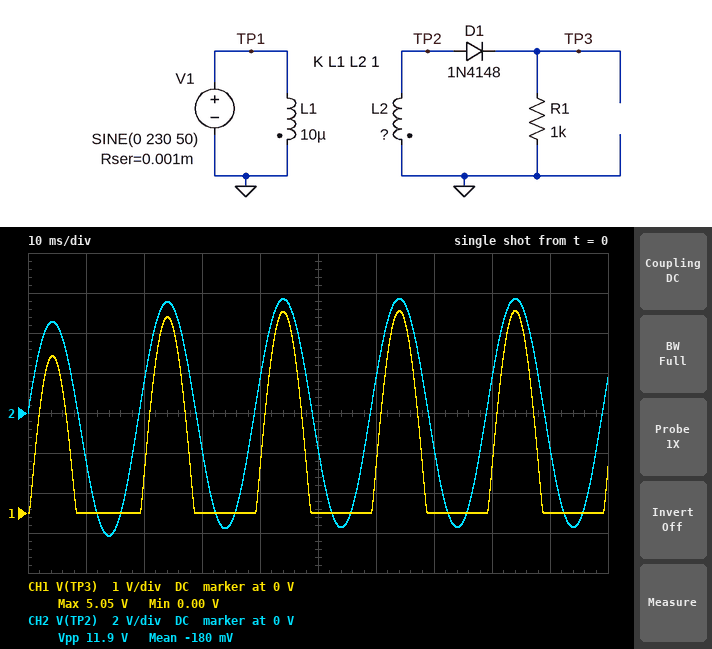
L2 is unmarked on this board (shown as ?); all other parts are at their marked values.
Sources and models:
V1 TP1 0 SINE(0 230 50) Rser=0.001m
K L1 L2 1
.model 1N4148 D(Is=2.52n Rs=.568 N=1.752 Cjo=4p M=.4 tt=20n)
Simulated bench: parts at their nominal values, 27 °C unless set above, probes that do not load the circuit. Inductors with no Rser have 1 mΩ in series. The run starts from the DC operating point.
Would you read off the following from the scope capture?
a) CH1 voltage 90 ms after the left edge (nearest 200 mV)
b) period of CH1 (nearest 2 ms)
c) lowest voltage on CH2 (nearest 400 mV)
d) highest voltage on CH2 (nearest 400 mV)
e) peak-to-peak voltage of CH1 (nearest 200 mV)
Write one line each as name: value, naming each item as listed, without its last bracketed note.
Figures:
CH1 voltage 90 ms after the left edge: 0 V
period of CH1: 20 ms
lowest voltage on CH2: -6.0 V
highest voltage on CH2: 5.6 V
peak-to-peak voltage of CH1: 5.0 V
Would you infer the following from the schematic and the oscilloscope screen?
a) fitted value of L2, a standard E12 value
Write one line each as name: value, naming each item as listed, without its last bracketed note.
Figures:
fitted value of L2, a standard E12 value: 6.8 nH
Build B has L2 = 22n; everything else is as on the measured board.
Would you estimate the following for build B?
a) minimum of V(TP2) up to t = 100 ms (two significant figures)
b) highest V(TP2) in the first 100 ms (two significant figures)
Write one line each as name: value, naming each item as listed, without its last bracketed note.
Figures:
minimum of V(TP2) up to t = 100 ms: -11 V
highest V(TP2) in the first 100 ms: 10 V
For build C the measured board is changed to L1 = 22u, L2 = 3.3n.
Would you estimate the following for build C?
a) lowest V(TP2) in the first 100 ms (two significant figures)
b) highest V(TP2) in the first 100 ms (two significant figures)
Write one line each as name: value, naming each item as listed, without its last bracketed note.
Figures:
lowest V(TP2) in the first 100 ms: -3.0 V
highest V(TP2) in the first 100 ms: 2.8 V
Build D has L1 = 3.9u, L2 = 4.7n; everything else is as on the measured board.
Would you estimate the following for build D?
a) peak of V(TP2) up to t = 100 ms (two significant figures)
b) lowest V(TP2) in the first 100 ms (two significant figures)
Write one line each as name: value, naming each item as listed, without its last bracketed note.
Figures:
peak of V(TP2) up to t = 100 ms: 6.2 V
lowest V(TP2) in the first 100 ms: -6.3 V
